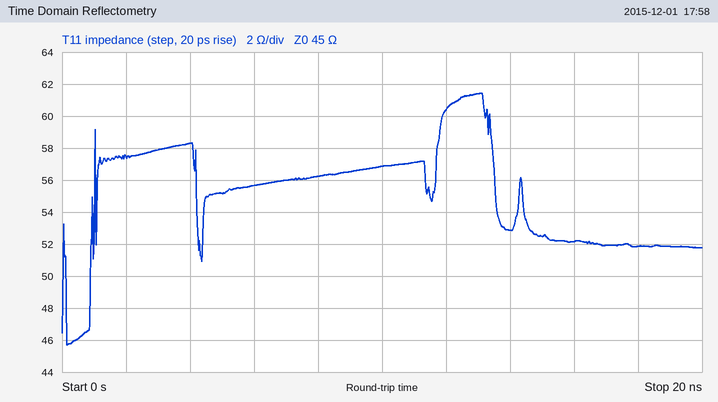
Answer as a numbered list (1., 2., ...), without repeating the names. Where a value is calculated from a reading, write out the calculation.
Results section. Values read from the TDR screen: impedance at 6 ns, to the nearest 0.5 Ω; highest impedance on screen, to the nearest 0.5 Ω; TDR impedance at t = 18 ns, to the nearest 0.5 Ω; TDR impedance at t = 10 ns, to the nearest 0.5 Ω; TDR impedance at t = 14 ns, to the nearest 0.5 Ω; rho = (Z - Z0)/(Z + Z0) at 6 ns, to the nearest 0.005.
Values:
1. 55.5 Ω
2. 61.5 Ω
3. 52.0 Ω
4. 57.0 Ω
5. 53.0 Ω
6. (55.5 − 45)/(55.5 + 45) ≈ +0.104, so +0.105 to the nearest 0.005
